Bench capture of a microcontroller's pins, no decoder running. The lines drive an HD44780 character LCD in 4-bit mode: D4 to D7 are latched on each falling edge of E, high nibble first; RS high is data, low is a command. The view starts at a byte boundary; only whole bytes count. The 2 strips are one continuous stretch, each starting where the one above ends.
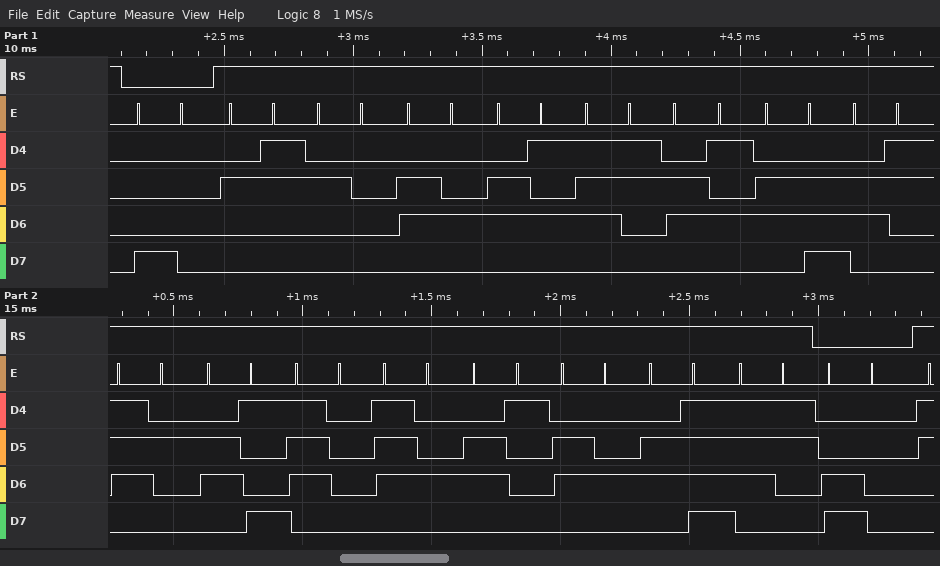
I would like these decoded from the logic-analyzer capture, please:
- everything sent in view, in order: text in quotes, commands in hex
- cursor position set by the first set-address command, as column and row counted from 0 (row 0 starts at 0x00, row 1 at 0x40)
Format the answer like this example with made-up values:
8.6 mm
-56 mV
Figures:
0x80 "# desencriptados" 0xC0
column 0, row 0
